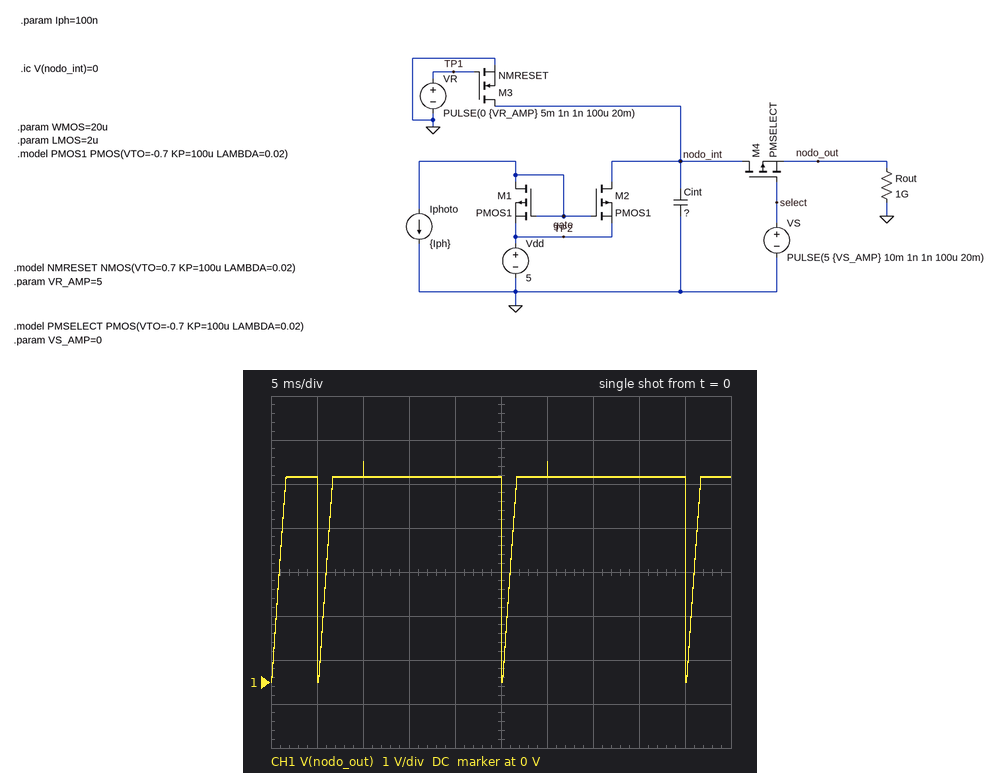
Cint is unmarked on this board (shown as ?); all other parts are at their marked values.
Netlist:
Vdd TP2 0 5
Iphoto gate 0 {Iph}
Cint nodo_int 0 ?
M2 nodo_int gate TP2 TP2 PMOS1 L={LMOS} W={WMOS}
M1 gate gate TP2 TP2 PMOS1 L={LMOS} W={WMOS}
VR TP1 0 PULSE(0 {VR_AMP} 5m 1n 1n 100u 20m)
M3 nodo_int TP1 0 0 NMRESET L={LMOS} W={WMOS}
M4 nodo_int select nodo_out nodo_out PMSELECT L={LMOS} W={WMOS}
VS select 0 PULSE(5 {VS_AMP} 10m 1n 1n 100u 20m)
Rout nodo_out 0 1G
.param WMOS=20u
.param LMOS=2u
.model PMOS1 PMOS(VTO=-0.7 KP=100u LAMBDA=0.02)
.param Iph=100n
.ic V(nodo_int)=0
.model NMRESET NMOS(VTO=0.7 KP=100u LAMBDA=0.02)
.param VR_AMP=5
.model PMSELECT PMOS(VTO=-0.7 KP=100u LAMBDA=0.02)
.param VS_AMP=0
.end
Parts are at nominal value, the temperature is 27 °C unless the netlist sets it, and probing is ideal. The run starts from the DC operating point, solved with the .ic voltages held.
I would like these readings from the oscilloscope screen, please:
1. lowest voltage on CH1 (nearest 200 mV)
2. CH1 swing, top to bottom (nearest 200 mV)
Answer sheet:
0 V
5.0 V
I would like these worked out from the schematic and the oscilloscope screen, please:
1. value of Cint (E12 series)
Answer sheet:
33 pF
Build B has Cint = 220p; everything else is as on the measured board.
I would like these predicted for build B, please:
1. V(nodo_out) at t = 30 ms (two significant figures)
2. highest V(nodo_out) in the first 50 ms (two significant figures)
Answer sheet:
2.0 V
4.7 V
